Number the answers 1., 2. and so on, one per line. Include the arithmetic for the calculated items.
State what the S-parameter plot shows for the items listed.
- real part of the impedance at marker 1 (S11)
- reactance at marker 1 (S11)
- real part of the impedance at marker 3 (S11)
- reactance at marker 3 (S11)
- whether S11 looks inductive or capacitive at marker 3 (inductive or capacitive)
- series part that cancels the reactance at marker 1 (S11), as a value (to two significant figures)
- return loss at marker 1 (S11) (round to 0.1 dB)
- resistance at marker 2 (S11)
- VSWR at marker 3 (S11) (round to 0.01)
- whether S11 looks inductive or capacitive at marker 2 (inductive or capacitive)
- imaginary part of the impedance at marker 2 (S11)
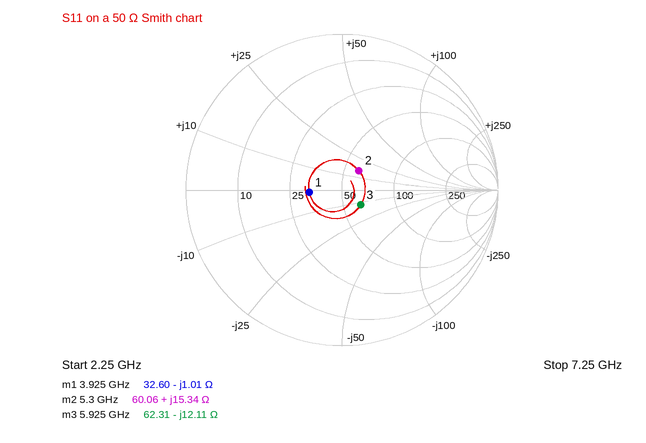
1. 32.60 Ω
2. -1.01 Ω
3. 62.31 Ω
4. -12.11 Ω
5. capacitive
6. L = 1.01 Ω/(2π × 3.925 GHz) ≈ 41 pH
7. 13.5 dB
8. 60.06 Ω
9. 1.36
10. inductive
11. +15.34 Ω
